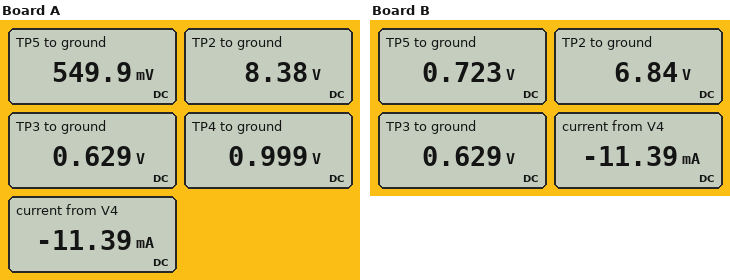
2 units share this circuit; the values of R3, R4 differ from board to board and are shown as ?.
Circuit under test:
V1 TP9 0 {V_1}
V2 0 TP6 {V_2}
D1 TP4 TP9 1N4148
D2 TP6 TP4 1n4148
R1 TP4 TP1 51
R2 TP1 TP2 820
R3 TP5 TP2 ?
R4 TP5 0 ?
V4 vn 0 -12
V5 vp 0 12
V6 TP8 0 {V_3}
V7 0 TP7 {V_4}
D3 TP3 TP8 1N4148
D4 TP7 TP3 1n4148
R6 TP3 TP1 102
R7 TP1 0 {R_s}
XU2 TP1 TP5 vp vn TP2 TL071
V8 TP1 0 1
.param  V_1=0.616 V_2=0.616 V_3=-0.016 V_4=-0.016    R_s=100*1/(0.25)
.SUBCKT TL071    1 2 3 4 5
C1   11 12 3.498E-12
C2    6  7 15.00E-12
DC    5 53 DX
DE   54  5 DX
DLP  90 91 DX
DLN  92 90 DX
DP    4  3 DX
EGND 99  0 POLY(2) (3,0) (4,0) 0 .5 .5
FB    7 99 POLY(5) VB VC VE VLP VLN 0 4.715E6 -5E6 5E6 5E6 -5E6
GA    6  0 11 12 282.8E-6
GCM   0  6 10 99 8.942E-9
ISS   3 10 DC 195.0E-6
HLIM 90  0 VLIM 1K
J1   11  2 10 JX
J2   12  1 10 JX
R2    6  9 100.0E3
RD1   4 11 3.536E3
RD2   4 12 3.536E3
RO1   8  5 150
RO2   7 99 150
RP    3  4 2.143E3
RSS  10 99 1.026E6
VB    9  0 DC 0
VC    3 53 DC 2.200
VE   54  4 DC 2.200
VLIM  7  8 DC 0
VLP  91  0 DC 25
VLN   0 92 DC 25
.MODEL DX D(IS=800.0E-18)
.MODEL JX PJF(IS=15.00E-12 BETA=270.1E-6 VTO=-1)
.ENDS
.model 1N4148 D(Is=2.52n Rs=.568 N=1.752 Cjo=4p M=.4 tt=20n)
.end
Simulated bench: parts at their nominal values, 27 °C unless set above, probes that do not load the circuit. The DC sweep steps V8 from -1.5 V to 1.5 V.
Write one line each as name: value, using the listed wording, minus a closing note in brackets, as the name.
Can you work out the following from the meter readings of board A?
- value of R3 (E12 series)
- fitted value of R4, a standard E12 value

value of R3: 470 Ω
fitted value of R4, a standard E12 value: 33 Ω
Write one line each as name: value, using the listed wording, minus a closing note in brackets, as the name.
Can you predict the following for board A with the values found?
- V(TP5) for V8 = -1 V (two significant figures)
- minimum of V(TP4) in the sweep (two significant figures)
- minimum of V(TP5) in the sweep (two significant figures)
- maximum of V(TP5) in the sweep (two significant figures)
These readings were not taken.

V(TP5) for V8 = -1 V: -550 mV
minimum of V(TP4) in the sweep: -1.3 V
minimum of V(TP5) in the sweep: -560 mV
maximum of V(TP5) in the sweep: 560 mV
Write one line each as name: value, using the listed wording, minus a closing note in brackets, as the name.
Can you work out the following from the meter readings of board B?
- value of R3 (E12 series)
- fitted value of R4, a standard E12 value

value of R3: 330 Ω
fitted value of R4, a standard E12 value: 39 Ω
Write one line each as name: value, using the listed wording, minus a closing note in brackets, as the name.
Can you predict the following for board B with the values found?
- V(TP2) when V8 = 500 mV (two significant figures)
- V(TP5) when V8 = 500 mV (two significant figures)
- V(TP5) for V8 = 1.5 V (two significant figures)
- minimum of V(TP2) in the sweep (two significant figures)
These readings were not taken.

V(TP2) when V8 = 500 mV: 4.7 V
V(TP5) when V8 = 500 mV: 500 mV
V(TP5) for V8 = 1.5 V: 740 mV
minimum of V(TP2) in the sweep: -7.0 V
